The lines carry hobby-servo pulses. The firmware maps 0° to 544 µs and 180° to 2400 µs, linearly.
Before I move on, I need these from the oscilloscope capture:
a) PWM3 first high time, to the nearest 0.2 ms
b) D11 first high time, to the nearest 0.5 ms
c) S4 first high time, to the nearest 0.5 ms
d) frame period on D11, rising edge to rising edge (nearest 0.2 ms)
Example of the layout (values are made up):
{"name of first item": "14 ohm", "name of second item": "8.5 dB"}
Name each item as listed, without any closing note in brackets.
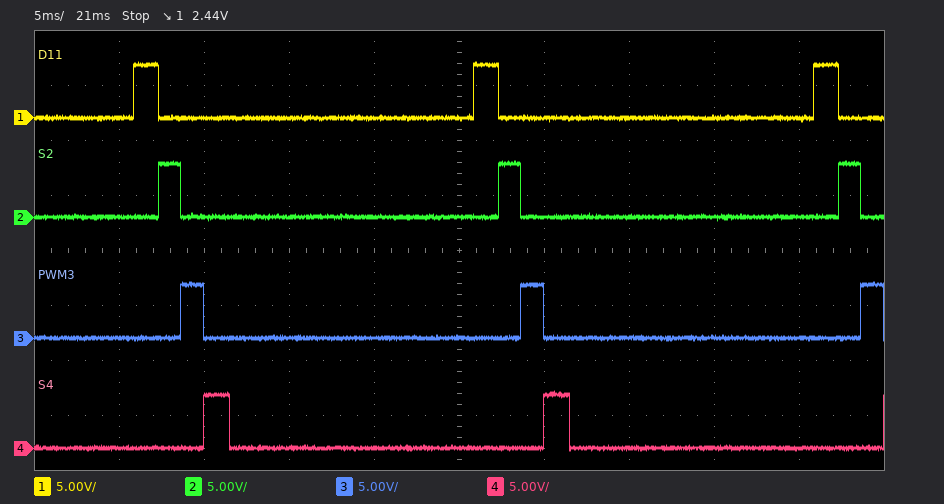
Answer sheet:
{"PWM3 first high time, to the nearest 0.2 ms": "1.4 ms", "D11 first high time, to the nearest 0.5 ms": "1.5 ms", "S4 first high time, to the nearest 0.5 ms": "1.5 ms", "frame period on D11, rising edge to rising edge": "20.0 ms"}
